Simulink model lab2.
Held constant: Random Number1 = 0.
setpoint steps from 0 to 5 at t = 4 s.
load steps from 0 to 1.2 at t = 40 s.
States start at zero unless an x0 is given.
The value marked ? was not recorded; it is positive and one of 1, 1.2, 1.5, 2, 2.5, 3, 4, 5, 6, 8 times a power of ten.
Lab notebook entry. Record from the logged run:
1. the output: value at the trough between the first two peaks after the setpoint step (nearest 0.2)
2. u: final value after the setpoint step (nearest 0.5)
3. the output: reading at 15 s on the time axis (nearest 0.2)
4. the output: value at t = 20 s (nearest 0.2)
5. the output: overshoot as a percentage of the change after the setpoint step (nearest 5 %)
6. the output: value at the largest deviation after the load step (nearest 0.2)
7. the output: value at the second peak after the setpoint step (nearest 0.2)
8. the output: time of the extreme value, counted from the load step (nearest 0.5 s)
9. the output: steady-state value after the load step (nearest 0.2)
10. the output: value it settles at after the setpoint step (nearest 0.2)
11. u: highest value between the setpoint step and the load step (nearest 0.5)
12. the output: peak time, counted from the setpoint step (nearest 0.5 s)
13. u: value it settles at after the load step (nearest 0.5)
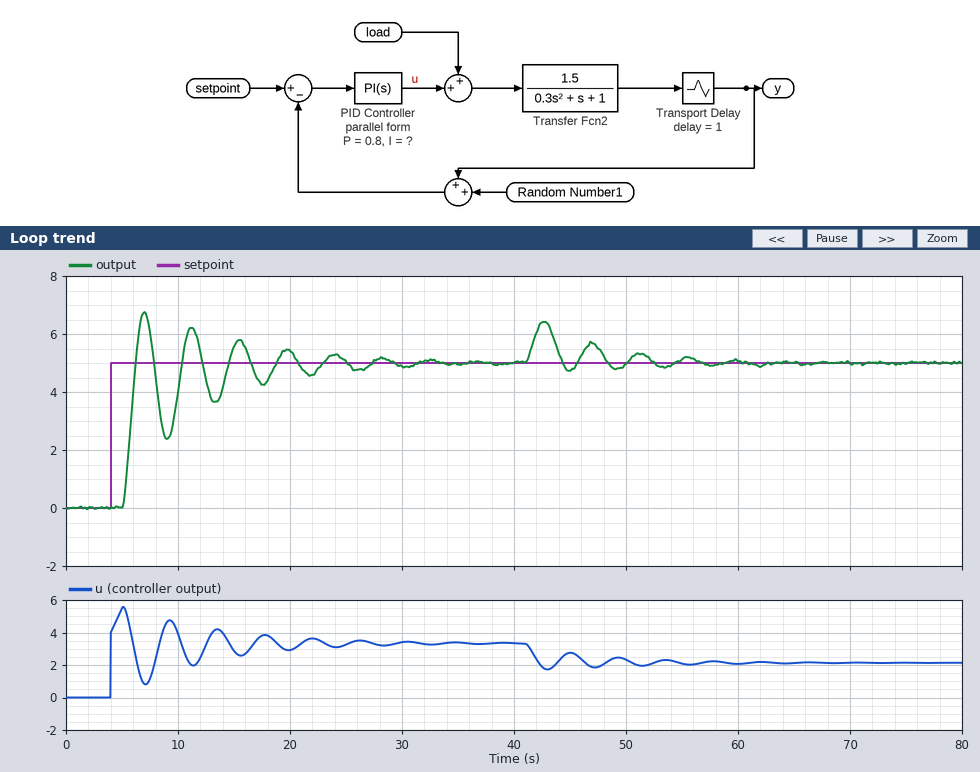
2.4
3.5
5.6
5.4
35 %
6.4
6.2
2.5 s
5.0
5.0
5.5
3.0 s
2.0
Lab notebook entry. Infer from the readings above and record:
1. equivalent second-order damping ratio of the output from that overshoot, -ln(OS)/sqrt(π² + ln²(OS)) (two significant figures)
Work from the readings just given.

0.32
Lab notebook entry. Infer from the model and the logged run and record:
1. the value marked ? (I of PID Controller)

0.3
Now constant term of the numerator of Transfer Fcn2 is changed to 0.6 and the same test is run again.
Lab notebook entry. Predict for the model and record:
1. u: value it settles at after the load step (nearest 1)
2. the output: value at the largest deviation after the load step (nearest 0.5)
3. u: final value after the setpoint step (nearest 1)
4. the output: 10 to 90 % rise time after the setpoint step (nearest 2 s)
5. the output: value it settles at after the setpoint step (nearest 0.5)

7
5.5
8
12 s
5.0
